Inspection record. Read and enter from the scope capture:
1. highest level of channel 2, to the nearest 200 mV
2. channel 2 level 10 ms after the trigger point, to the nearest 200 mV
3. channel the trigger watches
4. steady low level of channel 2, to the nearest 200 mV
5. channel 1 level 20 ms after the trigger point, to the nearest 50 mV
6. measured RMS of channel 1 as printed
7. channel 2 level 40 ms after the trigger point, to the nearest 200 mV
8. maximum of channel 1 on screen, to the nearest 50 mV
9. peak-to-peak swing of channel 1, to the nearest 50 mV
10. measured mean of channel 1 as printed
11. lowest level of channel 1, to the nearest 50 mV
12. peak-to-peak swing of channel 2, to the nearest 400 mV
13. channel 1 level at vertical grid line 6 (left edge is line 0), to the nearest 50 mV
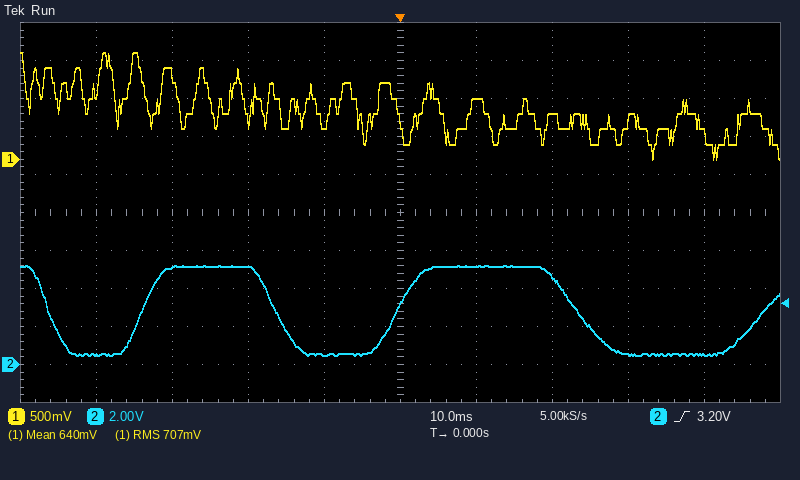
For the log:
5.2 V
5.2 V
channel 2
600 mV
600 mV
707 mV
600 mV
1.40 V
1.40 V
640 mV
0 mV
4.8 V
800 mV
